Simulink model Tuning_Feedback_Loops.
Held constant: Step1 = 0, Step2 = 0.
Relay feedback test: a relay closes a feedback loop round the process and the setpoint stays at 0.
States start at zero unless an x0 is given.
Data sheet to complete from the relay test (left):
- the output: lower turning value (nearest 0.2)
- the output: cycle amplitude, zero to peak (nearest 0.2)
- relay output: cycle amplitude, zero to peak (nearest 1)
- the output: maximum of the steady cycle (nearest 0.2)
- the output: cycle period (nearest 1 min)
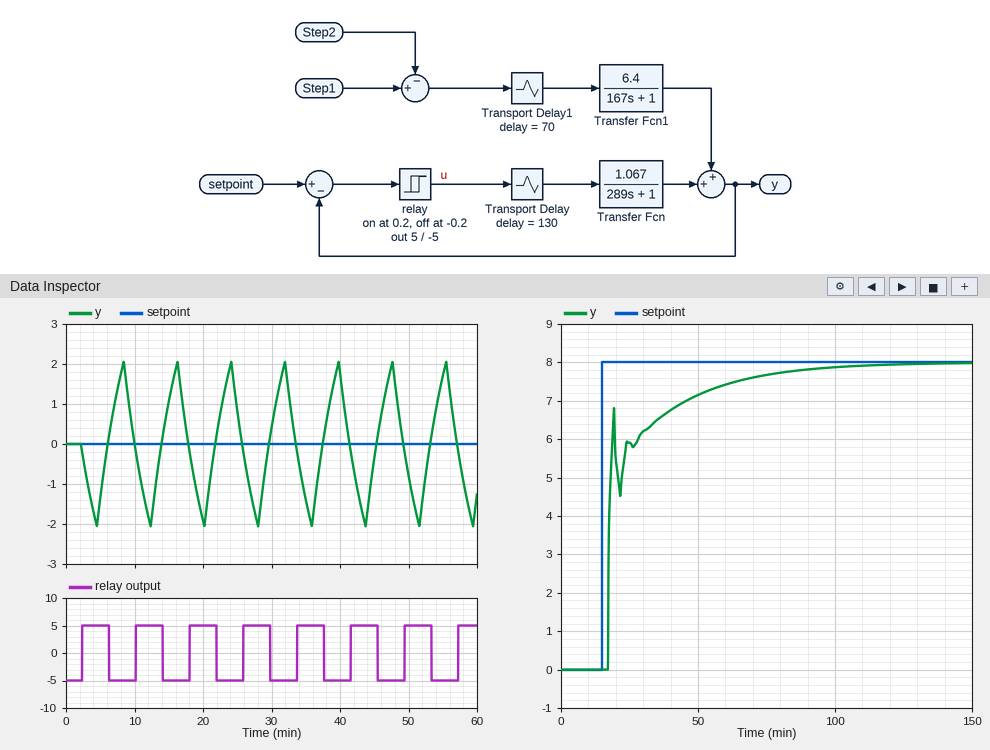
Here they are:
-2.0
2.0
5
2.0
8 min
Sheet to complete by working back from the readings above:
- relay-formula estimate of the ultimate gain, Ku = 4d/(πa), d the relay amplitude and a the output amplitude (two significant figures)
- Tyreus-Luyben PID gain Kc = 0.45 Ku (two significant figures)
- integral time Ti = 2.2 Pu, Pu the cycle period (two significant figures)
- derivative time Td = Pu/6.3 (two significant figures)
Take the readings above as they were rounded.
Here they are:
3.2
1.4
18 min
1.3 min
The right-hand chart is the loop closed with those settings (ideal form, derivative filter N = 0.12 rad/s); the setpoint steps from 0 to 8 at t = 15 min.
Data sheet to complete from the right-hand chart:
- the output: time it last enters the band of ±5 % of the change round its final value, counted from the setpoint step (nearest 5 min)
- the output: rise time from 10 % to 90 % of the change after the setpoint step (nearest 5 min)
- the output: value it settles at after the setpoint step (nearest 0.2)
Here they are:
55 min
35 min
8.0
